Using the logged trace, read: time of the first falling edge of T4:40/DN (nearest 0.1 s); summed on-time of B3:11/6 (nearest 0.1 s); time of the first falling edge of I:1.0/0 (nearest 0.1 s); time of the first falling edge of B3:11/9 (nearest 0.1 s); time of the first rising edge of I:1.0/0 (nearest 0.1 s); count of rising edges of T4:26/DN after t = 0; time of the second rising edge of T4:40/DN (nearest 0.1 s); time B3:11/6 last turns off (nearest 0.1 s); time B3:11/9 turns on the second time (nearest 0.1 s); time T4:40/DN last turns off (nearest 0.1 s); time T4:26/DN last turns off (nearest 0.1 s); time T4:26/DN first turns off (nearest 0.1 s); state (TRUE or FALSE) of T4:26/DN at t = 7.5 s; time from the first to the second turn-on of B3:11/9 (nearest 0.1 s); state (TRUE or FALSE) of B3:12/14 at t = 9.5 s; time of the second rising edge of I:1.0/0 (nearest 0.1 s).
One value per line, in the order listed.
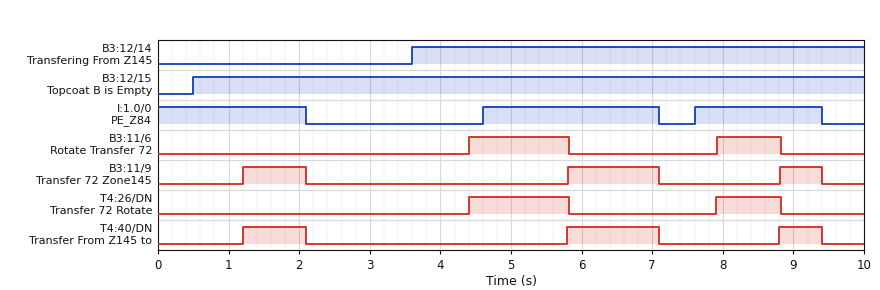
2.1 s
2.3 s
2.1 s
2.1 s
4.6 s
2
5.8 s
8.8 s
5.8 s
9.4 s
8.8 s
5.8 s
FALSE
4.6 s
TRUE
7.6 s
